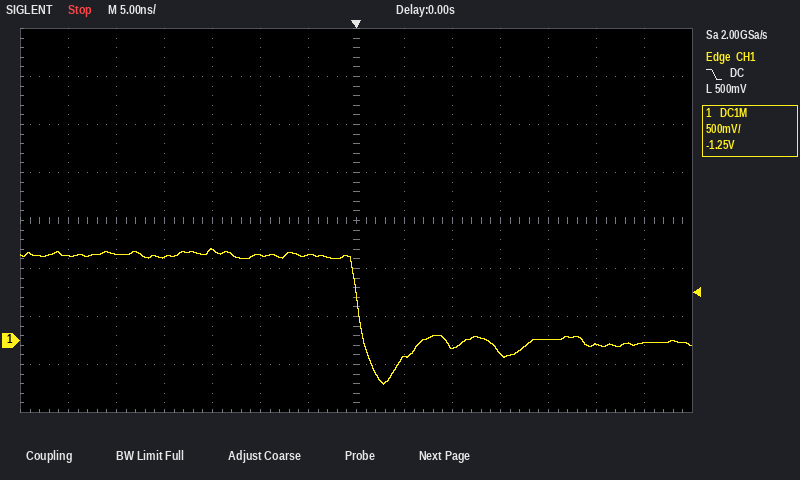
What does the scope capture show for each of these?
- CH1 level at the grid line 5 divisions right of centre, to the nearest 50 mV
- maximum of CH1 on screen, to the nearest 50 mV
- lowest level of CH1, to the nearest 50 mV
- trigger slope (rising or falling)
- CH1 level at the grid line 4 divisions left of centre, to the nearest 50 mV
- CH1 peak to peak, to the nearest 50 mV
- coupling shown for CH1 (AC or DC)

-50 mV
950 mV
-450 mV
falling
850 mV
1.40 V
DC
